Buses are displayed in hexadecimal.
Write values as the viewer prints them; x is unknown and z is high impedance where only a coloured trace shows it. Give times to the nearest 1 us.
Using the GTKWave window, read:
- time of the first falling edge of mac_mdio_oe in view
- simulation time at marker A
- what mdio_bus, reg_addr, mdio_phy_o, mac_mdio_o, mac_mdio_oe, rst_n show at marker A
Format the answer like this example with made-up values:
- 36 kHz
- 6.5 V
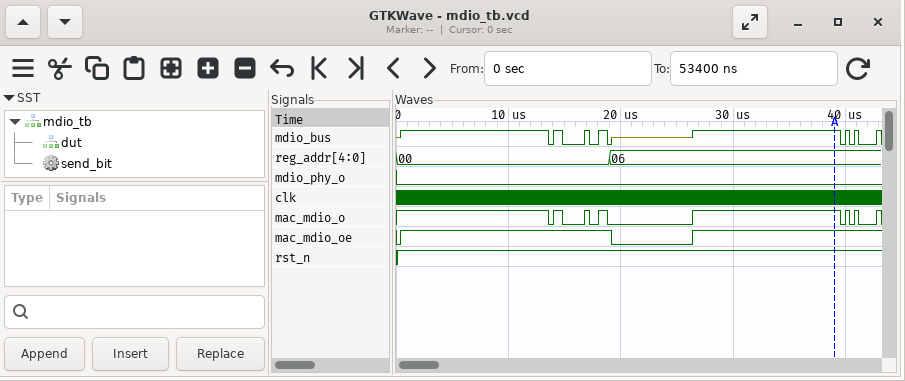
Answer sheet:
- 19 us
- 39 us
- mdio_bus=1, reg_addr=06, mdio_phy_o=0, mac_mdio_o=1, mac_mdio_oe=1, rst_n=1
